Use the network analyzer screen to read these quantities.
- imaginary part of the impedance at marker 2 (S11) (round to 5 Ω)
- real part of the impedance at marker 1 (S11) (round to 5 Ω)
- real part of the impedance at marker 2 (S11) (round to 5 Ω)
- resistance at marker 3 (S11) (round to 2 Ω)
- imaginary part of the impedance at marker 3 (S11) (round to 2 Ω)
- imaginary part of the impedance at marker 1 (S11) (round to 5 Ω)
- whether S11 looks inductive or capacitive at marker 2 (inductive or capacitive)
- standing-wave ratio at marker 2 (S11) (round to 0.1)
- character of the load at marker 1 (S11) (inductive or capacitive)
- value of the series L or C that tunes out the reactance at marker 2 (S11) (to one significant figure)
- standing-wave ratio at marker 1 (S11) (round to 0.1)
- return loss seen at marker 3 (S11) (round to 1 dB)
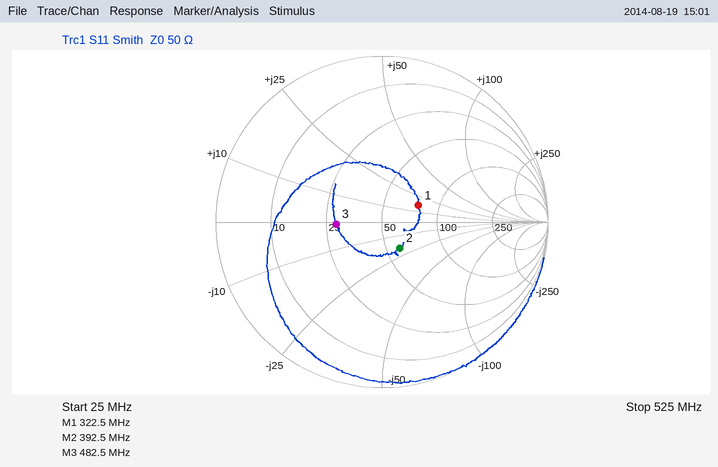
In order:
-20 Ω
75 Ω
60 Ω
28 Ω
0 Ω
+15 Ω
capacitive
1.5
inductive
8 nH
1.6
11 dB
